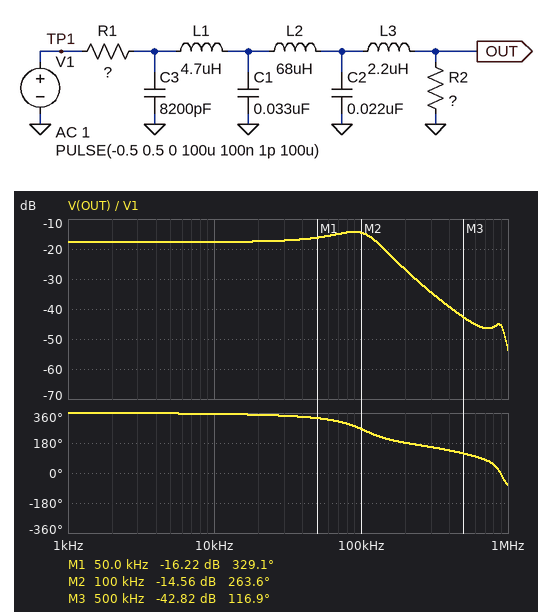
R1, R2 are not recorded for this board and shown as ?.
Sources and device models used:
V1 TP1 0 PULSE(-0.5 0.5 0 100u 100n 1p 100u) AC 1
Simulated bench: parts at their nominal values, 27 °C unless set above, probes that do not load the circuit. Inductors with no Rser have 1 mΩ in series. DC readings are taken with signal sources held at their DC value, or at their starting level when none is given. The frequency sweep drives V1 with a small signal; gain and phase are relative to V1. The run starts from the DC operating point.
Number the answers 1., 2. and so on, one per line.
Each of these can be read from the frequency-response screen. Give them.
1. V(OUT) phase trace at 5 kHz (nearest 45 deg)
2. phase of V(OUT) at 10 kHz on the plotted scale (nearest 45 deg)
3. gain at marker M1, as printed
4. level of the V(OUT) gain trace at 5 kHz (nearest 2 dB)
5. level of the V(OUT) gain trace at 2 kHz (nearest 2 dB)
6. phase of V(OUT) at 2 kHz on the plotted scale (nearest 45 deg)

1. 360 deg
2. 360 deg
3. -16.22 dB
4. -18 dB
5. -18 dB
6. 360 deg
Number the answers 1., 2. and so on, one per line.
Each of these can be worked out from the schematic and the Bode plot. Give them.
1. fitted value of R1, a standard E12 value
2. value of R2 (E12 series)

1. 100 Ω
2. 15 Ω
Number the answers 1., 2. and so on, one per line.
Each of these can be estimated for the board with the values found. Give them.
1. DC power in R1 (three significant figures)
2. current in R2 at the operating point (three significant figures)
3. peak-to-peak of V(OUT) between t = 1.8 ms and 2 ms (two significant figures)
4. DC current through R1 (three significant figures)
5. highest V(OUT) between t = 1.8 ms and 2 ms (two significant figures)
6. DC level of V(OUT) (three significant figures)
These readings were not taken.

1. 1.89 mW
2. 4.35 mA
3. 160 mV
4. 4.35 mA
5. 64 mV
6. -65.2 mV
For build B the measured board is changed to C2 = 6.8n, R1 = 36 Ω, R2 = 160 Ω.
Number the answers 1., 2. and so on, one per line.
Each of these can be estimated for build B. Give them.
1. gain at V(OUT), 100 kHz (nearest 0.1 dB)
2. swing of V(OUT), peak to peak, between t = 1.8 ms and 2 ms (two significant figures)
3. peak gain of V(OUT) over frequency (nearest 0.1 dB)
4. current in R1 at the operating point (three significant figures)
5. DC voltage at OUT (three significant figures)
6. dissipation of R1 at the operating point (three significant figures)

1. -2.8 dB
2. 820 mV
3. -1.8 dB
4. 2.55 mA
5. -408 mV
6. 234 µW
